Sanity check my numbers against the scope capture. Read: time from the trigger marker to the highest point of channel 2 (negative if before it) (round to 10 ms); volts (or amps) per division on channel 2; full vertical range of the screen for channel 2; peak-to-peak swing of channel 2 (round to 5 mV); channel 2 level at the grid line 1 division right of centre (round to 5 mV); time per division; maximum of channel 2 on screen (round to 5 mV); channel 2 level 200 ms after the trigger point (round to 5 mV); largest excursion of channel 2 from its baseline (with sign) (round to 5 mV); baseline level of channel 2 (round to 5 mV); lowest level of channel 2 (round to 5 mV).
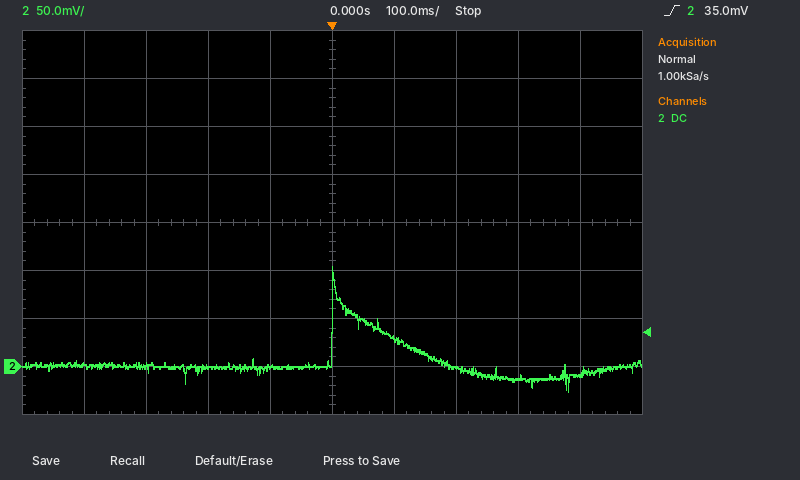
0 ms
50 mV
400 mV
130 mV
30 mV
100 ms
105 mV
0 mV
+105 mV
0 mV
-25 mV
